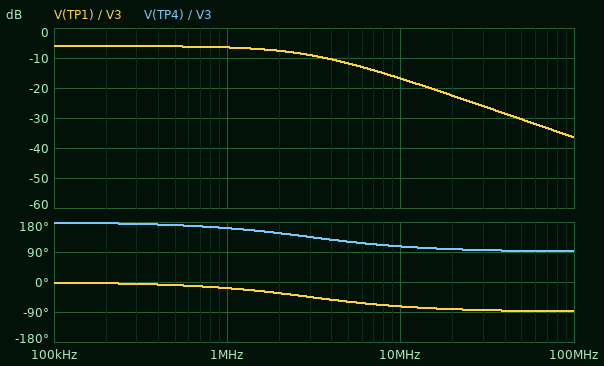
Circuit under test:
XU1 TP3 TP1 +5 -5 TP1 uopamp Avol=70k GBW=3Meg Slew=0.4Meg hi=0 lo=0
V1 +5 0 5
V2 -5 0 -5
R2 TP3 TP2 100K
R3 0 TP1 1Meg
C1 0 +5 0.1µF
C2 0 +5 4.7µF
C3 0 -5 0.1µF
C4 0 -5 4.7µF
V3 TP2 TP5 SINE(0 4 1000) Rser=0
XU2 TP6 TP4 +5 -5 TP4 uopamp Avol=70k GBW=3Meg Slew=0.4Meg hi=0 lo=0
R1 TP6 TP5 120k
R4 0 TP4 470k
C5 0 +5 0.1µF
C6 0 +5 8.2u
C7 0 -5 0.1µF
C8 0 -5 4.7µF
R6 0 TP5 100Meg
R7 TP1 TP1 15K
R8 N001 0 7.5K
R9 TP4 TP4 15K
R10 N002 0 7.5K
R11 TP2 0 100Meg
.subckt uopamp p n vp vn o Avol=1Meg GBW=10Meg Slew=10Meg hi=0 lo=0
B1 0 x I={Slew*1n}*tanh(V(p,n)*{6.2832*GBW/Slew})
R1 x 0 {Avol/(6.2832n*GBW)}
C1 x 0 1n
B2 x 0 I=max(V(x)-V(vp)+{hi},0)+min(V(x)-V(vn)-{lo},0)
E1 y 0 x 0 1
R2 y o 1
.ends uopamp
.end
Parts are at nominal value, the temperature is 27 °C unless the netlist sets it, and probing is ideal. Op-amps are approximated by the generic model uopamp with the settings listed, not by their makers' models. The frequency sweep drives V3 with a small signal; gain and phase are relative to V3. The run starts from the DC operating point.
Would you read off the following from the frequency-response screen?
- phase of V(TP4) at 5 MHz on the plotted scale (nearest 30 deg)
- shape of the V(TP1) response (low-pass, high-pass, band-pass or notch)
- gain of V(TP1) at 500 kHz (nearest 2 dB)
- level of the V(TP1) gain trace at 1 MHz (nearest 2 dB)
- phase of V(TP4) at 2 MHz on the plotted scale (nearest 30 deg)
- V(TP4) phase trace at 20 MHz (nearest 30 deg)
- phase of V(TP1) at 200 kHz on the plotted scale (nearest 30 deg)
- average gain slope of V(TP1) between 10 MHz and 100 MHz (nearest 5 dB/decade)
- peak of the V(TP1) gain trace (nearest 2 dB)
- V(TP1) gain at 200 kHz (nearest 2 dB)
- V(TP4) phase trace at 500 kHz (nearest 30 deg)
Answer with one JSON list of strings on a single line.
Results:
["120 deg", "low-pass", "-6 dB", "-6 dB", "150 deg", "90 deg", "0 deg", "-20 dB/decade", "-6 dB", "-6 dB", "180 deg"]
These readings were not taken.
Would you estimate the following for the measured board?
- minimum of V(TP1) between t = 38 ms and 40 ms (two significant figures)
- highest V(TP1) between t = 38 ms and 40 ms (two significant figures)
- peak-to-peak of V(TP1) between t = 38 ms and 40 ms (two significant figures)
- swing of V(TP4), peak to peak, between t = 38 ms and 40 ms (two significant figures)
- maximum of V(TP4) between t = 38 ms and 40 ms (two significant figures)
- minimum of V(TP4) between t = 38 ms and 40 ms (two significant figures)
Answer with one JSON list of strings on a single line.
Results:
["-2.0 V", "2.0 V", "4.0 V", "4.0 V", "2.0 V", "-2.0 V"]
